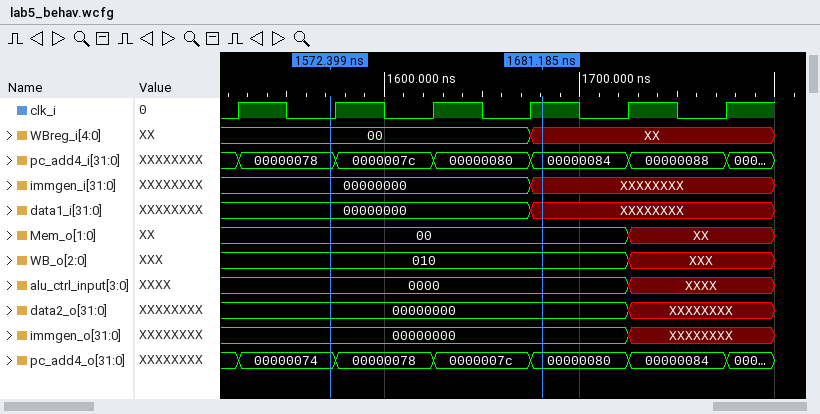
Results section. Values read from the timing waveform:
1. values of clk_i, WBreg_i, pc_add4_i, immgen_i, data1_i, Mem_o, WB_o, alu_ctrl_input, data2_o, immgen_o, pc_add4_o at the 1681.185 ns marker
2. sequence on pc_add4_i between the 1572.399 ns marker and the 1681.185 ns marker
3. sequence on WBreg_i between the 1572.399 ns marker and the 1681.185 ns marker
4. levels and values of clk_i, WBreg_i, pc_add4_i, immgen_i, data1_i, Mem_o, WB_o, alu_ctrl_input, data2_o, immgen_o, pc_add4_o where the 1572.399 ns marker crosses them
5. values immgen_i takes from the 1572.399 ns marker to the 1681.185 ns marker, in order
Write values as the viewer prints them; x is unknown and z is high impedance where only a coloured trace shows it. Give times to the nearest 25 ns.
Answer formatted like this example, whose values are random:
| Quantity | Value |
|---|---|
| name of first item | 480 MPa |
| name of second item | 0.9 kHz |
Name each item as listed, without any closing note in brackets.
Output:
| Quantity | Value |
|---|---|
| values of clk_i, WBreg_i, pc_add4_i, immgen_i, data1_i, Mem_o, WB_o, alu_ctrl_input, data2_o, immgen_o, pc_add4_o at the 1681.185 ns marker | clk_i=1, WBreg_i=XX, pc_add4_i=00000084, immgen_i=XXXXXXXX, data1_i=XXXXXXXX, Mem_o=00, WB_o=010, alu_ctrl_input=0000, data2_o=00000000, immgen_o=00000000, pc_add4_o=00000080 |
| sequence on pc_add4_i between the 1572.399 ns marker and the 1681.185 ns marker | 00000078, 0000007c, 00000080, 00000084 |
| sequence on WBreg_i between the 1572.399 ns marker and the 1681.185 ns marker | 00, XX |
| levels and values of clk_i, WBreg_i, pc_add4_i, immgen_i, data1_i, Mem_o, WB_o, alu_ctrl_input, data2_o, immgen_o, pc_add4_o where the 1572.399 ns marker crosses them | clk_i=0, WBreg_i=00, pc_add4_i=00000078, immgen_i=00000000, data1_i=00000000, Mem_o=00, WB_o=010, alu_ctrl_input=0000, data2_o=00000000, immgen_o=00000000, pc_add4_o=00000074 |
| values immgen_i takes from the 1572.399 ns marker to the 1681.185 ns marker, in order | 00000000, XXXXXXXX |
